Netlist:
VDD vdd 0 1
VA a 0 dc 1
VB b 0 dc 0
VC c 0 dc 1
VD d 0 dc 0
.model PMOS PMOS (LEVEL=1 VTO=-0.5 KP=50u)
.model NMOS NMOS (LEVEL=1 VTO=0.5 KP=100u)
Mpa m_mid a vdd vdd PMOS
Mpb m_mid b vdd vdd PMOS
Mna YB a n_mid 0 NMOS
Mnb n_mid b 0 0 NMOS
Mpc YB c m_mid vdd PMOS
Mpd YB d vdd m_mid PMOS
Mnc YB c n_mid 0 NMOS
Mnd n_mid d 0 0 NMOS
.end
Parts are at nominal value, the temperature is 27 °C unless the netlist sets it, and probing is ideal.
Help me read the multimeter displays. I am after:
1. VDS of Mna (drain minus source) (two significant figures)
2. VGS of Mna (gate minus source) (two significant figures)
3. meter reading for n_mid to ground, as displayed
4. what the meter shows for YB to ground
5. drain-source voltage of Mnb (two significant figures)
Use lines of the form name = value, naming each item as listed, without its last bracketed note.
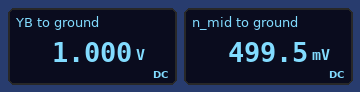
VDS of Mna (drain minus source) = 500 mV
VGS of Mna (gate minus source) = 500 mV
meter reading for n_mid to ground, as displayed = 499.5 mV
what the meter shows for YB to ground = 1.000 V
drain-source voltage of Mnb = 500 mV
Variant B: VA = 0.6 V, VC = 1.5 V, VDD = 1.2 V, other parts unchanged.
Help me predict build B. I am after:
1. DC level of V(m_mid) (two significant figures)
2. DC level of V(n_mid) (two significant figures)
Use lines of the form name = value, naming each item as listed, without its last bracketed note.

DC level of V(m_mid) = 1.2 V
DC level of V(n_mid) = 1.0 V
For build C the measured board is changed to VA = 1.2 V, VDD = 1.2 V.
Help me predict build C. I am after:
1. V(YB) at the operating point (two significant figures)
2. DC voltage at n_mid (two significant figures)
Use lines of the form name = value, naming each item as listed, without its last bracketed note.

V(YB) at the operating point = 1.2 V
DC voltage at n_mid = 700 mV
